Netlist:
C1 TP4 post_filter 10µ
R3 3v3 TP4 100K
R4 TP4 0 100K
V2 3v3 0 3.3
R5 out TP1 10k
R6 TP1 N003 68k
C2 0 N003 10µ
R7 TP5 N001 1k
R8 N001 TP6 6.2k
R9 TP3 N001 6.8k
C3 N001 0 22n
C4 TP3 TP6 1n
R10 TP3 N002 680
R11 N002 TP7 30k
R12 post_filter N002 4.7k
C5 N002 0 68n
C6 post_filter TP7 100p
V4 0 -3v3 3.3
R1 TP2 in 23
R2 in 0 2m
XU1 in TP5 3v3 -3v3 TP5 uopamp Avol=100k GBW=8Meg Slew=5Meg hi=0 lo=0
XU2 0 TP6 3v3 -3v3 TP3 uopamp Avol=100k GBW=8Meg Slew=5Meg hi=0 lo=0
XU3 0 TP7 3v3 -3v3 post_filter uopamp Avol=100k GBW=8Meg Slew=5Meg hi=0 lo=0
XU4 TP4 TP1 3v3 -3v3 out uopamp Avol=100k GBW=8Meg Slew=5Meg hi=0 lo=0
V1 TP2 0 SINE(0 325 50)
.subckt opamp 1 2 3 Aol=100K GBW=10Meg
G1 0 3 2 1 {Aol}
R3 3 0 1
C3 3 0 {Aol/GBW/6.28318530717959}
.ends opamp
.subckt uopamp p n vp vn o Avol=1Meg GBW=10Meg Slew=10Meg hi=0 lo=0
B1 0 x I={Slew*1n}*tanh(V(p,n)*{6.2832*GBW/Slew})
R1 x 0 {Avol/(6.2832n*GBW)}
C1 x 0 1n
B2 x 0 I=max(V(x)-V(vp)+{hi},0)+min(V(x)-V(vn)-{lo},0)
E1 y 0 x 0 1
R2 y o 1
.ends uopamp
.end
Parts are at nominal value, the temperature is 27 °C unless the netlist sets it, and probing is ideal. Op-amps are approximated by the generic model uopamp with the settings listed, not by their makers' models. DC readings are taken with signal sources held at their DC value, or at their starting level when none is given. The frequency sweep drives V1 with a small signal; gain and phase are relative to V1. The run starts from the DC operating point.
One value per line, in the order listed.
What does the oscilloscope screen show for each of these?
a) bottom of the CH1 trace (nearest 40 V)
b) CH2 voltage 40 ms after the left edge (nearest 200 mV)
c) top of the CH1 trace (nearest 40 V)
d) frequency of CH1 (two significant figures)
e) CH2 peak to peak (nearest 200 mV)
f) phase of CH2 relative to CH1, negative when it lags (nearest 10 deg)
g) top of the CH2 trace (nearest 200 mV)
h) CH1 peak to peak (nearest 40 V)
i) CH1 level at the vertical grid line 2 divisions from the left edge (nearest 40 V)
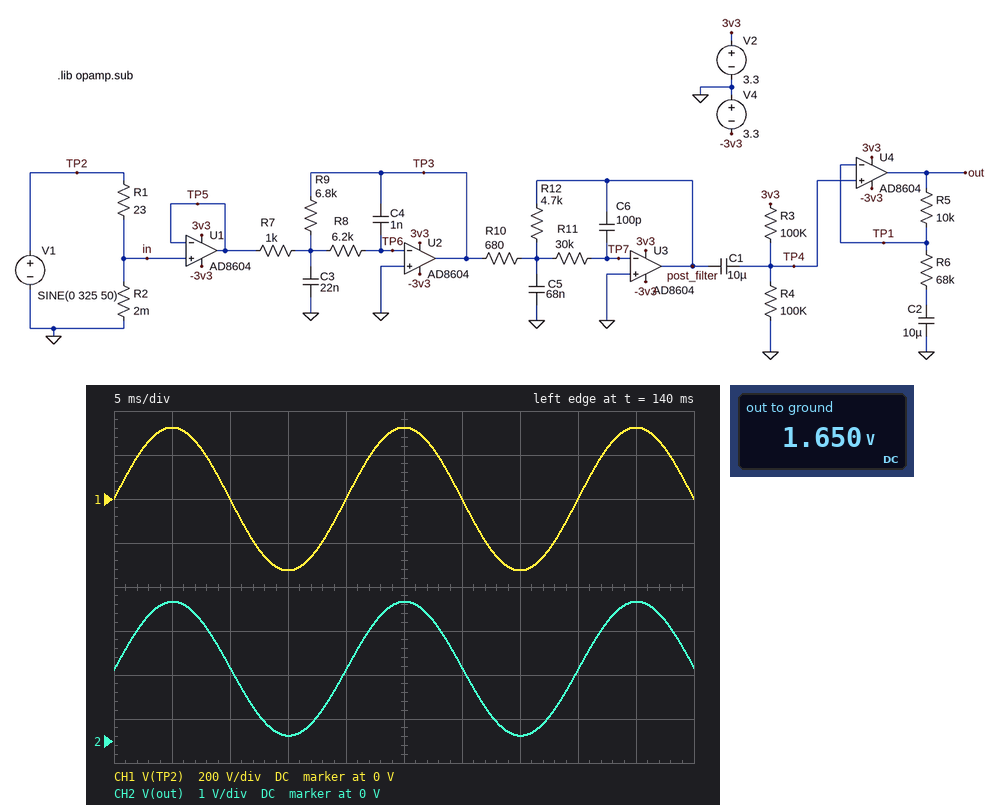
-320 V
1.6 V
320 V
50 Hz
3.0 V
0 deg
3.2 V
640 V
0 V
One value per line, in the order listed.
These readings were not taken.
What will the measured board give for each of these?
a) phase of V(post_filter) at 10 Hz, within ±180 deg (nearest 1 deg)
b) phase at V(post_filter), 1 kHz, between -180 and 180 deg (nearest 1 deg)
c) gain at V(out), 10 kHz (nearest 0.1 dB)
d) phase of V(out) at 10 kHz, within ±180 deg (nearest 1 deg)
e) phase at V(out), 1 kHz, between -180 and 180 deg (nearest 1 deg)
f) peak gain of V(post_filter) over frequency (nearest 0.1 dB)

0 deg
-29 deg
-69.5 dB
81 deg
-29 deg
-47.7 dB
